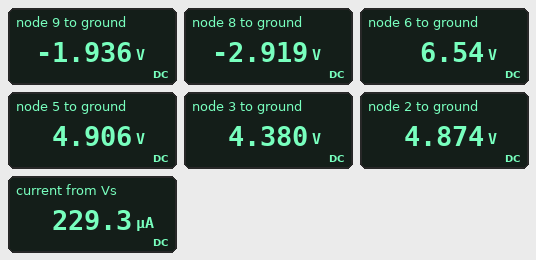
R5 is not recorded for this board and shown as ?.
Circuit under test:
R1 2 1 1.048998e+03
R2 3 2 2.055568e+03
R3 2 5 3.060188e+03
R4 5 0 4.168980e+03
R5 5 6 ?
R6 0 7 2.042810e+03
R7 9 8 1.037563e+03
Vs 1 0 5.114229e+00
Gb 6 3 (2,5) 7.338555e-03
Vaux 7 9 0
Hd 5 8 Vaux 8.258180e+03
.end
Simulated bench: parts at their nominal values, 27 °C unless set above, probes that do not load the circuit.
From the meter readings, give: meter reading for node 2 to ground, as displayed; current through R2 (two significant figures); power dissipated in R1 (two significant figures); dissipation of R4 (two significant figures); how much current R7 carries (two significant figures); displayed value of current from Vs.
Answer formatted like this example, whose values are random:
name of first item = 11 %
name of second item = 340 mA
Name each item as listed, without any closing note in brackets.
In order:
meter reading for node 2 to ground, as displayed = 4.874 V
current through R2 = 240 µA
power dissipated in R1 = 55 µW
dissipation of R4 = 5.8 mW
how much current R7 carries = 950 µA
displayed value of current from Vs = 229.3 µA
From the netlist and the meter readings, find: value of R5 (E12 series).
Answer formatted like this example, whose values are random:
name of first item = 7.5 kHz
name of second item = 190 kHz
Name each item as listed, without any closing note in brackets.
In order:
value of R5 = 6.8 kΩ
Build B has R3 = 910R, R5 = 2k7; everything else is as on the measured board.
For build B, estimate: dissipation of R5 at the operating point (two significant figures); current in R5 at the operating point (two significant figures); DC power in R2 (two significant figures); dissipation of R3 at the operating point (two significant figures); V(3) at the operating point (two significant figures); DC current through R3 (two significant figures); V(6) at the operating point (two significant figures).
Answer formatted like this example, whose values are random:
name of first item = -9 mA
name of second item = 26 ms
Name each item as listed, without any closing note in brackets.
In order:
dissipation of R5 at the operating point = 200 µW
current in R5 at the operating point = 270 µA
DC power in R2 = 150 µW
dissipation of R3 at the operating point = 1.5 µW
V(3) at the operating point = 4.3 V
DC current through R3 = 40 µA
V(6) at the operating point = 5.6 V
